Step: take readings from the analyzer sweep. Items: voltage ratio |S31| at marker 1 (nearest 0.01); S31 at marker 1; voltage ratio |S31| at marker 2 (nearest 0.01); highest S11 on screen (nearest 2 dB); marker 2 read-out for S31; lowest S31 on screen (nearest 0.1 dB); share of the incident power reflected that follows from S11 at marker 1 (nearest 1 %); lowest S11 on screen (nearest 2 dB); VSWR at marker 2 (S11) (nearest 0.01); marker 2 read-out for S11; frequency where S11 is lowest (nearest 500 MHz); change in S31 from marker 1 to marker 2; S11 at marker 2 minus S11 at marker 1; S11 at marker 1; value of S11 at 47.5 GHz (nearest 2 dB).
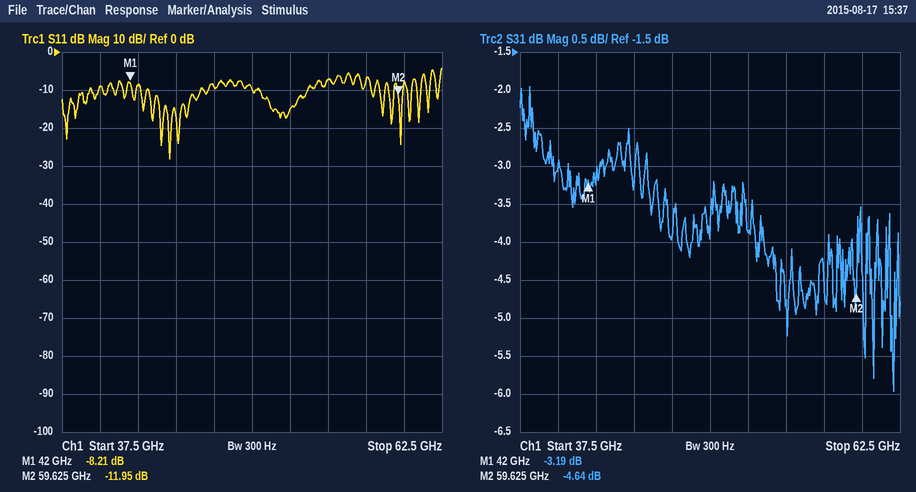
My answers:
0.69
-3.19 dB
0.59
-4 dB
-4.64 dB
-6.0 dB
15 %
-28 dB
1.68
-11.95 dB
44.5 GHz
-1.45 dB
-3.74 dB
-8.21 dB
-10 dB
